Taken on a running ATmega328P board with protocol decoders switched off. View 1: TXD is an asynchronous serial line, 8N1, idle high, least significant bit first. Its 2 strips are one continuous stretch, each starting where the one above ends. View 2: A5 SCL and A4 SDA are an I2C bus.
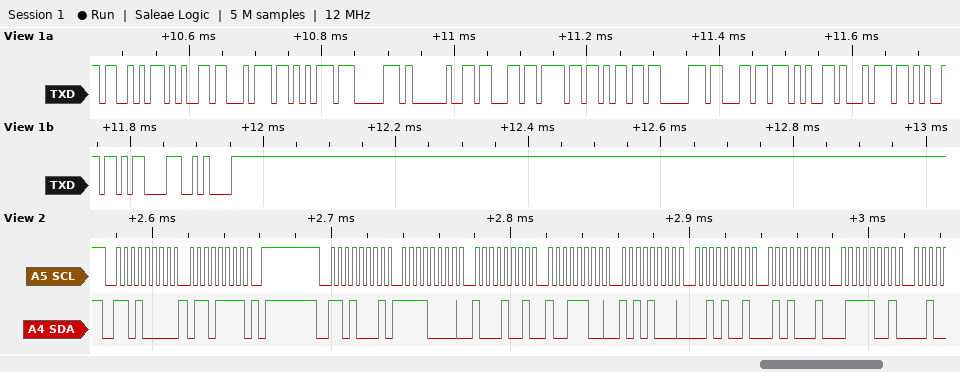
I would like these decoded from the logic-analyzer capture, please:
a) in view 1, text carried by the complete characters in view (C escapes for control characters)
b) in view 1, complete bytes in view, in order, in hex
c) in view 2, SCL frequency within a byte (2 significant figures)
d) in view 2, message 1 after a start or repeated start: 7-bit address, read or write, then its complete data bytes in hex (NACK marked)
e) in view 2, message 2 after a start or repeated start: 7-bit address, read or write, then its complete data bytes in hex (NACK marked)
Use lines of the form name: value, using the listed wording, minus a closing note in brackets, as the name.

in view 1, text carried by the complete characters in view: "Setup complete\r\n"
in view 1, complete bytes in view, in order, in hex: 0x53 0x65 0x74 0x75 0x70 0x20 0x63 0x6F 0x6D 0x70 0x6C 0x65 0x74 0x65 0x0D 0x0A
in view 2, SCL frequency within a byte: 250 kHz
in view 2, message 1 after a start or repeated start: 7-bit address, read or write, then its complete data bytes in hex: 0x68 write: 6F
in view 2, message 2 after a start or repeated start: 7-bit address, read or write, then its complete data bytes in hex: 0x68 read: F0 89 9C A8 29 51 79
